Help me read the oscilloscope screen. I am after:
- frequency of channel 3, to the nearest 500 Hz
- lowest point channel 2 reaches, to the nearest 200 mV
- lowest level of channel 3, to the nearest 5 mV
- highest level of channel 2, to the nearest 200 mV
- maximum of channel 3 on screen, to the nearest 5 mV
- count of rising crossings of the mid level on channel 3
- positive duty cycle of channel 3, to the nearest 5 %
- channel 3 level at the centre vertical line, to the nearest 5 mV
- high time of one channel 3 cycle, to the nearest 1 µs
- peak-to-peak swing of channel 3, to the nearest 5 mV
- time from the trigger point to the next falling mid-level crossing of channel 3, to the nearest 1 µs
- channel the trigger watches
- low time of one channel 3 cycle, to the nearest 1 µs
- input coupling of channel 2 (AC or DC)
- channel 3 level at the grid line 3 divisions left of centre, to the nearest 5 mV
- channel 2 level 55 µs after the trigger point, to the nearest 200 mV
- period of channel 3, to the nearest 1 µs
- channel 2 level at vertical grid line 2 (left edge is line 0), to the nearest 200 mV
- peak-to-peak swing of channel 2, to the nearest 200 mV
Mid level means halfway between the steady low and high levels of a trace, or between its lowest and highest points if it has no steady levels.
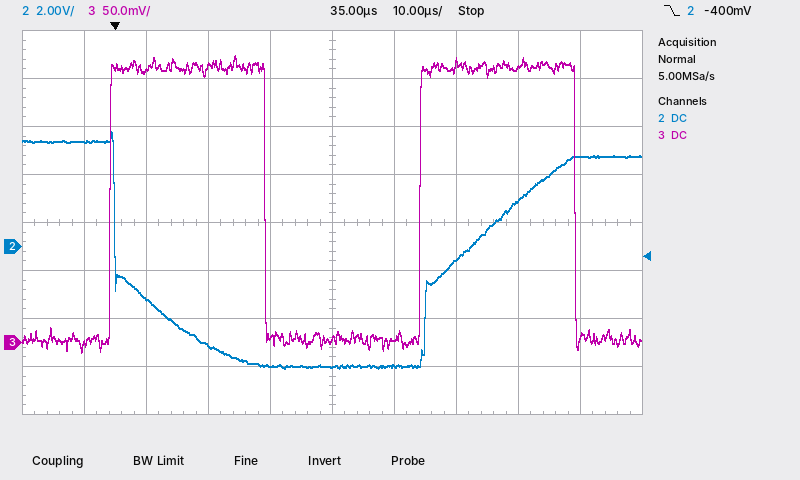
20.0 kHz
-5.0 V
-10 mV
4.8 V
300 mV
2
50 %
5 mV
25 µs
310 mV
24 µs
channel 2
25 µs
DC
285 mV
-600 mV
50 µs
-2.2 V
9.8 V
